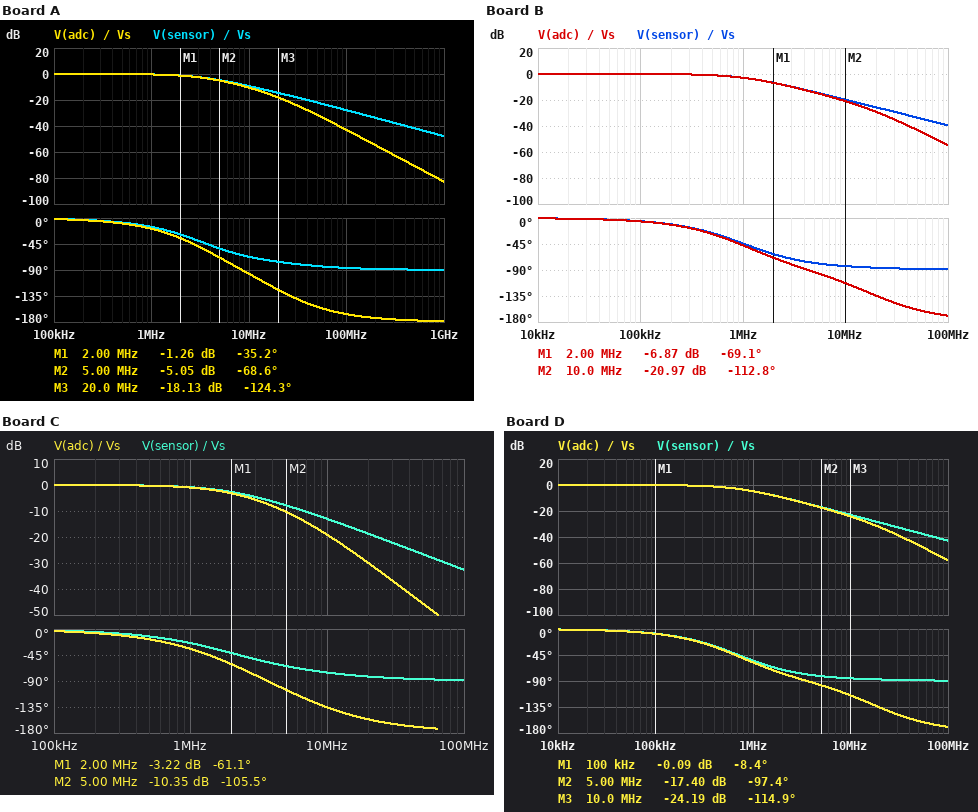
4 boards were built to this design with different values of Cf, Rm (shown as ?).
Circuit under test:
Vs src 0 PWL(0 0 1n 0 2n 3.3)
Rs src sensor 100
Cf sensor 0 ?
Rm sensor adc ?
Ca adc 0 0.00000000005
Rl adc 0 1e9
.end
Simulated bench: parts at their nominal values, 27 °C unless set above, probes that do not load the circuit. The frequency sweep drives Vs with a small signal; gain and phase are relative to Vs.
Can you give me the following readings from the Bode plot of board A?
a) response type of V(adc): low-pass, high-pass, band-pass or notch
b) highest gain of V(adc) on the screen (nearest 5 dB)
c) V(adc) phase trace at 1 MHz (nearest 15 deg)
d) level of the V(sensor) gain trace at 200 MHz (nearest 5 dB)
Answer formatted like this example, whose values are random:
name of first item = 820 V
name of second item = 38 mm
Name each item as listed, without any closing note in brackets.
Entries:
response type of V(adc): low-pass, high-pass, band-pass or notch = low-pass
highest gain of V(adc) on the screen = 0 dB
V(adc) phase trace at 1 MHz = -15 deg
level of the V(sensor) gain trace at 200 MHz = -35 dB
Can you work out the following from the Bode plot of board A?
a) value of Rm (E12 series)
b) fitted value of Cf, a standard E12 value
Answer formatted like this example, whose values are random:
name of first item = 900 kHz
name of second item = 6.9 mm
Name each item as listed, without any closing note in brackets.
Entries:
value of Rm = 180 Ω
fitted value of Cf, a standard E12 value = 390 pF
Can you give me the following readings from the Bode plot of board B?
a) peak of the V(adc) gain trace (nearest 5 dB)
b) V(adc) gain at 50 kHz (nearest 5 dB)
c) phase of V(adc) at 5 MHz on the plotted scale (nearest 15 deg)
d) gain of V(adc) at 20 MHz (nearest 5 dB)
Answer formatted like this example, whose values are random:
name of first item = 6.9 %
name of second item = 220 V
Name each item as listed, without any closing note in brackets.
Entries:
peak of the V(adc) gain trace = 0 dB
V(adc) gain at 50 kHz = 0 dB
phase of V(adc) at 5 MHz on the plotted scale = -90 deg
gain of V(adc) at 20 MHz = -30 dB
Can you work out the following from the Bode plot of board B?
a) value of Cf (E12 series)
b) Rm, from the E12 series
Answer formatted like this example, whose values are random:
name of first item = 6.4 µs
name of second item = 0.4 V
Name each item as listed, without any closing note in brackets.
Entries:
value of Cf = 1.5 nF
Rm, from the E12 series = 180 Ω
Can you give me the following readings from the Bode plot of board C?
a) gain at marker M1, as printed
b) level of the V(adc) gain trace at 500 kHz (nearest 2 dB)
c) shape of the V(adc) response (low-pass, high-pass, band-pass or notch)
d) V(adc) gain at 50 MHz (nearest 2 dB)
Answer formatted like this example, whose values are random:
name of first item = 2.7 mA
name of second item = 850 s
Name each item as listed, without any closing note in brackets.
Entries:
gain at marker M1, as printed = -3.22 dB
level of the V(adc) gain trace at 500 kHz = 0 dB
shape of the V(adc) response = low-pass
V(adc) gain at 50 MHz = -46 dB
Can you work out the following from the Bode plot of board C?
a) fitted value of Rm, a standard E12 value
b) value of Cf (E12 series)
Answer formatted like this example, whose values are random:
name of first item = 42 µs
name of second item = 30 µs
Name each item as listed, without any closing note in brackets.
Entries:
fitted value of Rm, a standard E12 value = 560 Ω
value of Cf = 680 pF
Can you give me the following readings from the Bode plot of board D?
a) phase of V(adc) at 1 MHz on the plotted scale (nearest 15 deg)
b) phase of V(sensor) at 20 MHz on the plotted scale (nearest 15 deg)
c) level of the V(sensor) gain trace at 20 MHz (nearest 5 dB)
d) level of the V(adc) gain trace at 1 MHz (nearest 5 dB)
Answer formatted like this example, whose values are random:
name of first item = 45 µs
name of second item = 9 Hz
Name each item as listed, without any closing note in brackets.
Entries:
phase of V(adc) at 1 MHz on the plotted scale = -60 deg
phase of V(sensor) at 20 MHz on the plotted scale = -90 deg
level of the V(sensor) gain trace at 20 MHz = -30 dB
level of the V(adc) gain trace at 1 MHz = -5 dB
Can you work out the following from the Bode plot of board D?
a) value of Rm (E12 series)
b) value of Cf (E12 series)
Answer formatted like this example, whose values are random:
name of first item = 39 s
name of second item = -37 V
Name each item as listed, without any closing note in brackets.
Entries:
value of Rm = 180 Ω
value of Cf = 2.2 nF
